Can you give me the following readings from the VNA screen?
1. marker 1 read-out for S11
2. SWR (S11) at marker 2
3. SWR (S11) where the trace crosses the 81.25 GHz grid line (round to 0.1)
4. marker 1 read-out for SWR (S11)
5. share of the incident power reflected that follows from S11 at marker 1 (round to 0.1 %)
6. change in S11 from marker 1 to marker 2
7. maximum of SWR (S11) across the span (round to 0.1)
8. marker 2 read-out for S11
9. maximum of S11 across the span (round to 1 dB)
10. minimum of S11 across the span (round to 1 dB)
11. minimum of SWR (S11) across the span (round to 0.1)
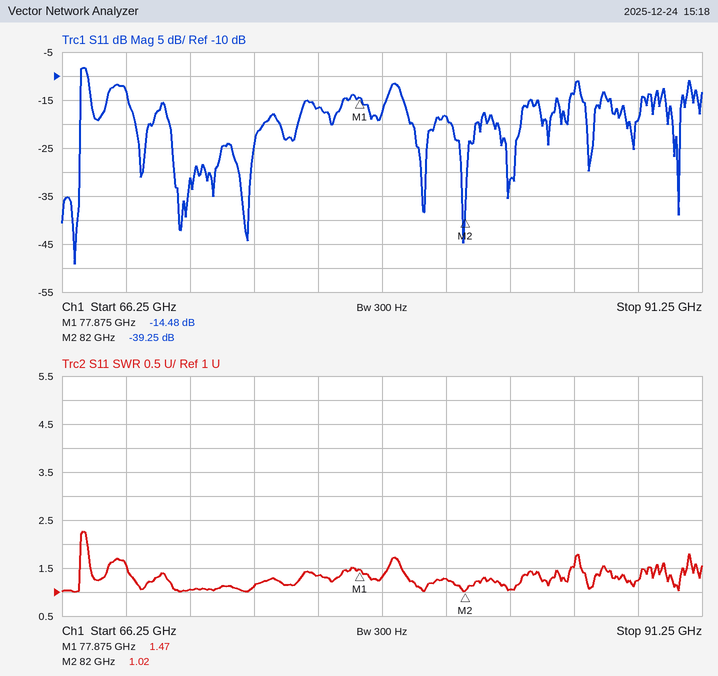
-14.48 dB
1.02
1.3
1.47
3.6 %
-24.77 dB
2.3
-39.25 dB
-8 dB
-49 dB
1.0
